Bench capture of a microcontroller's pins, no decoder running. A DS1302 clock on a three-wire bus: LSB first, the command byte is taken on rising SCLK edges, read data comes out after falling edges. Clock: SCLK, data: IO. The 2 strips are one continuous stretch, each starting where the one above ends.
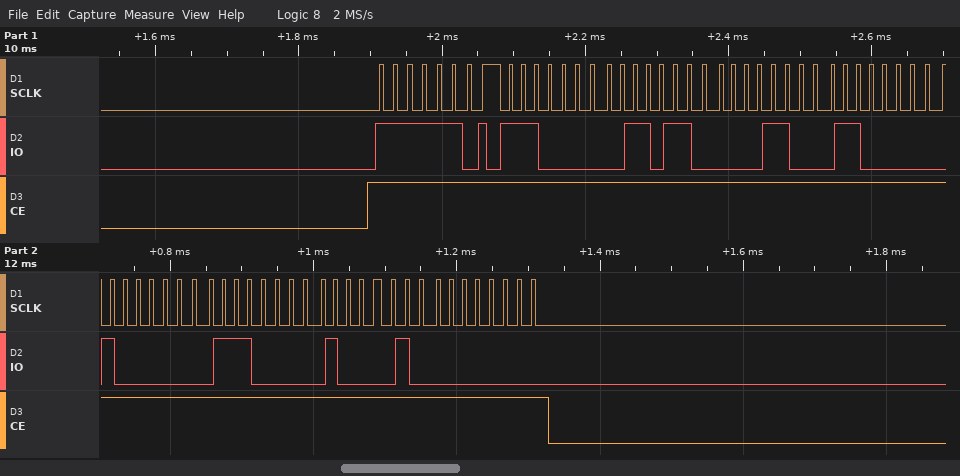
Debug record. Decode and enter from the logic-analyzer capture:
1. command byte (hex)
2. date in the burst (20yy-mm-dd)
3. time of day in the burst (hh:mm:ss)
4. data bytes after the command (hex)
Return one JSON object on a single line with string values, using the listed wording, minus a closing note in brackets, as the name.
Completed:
{"command byte": "0xBF", "date in the burst": "2021-01-03", "time of day in the burst": "18:36:07", "data bytes after the command": "07 36 18 03 01 07 21 00"}
